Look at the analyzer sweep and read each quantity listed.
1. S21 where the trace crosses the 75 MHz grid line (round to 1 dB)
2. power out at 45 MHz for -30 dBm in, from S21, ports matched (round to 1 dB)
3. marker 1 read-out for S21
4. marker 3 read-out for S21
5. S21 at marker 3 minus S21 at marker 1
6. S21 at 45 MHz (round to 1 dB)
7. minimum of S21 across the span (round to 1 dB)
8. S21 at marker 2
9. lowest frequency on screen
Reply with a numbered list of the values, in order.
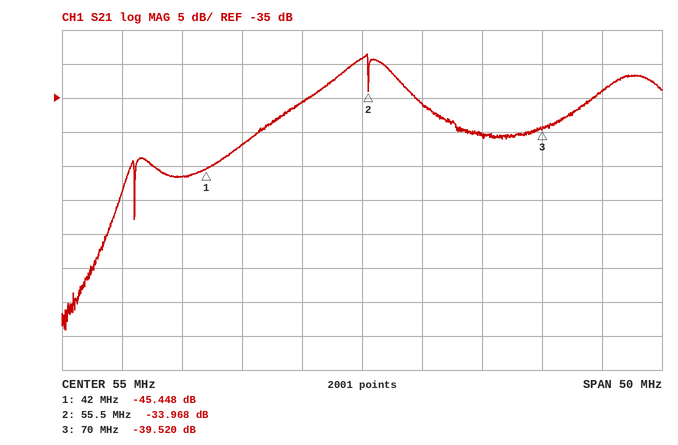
1. -34 dB
2. -72 dBm
3. -45.448 dB
4. -39.520 dB
5. 5.928 dB
6. -42 dB
7. -69 dB
8. -33.968 dB
9. 30 MHz
